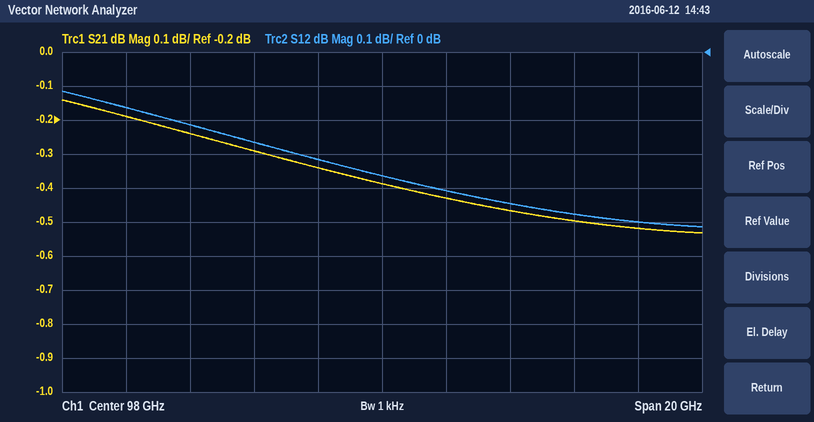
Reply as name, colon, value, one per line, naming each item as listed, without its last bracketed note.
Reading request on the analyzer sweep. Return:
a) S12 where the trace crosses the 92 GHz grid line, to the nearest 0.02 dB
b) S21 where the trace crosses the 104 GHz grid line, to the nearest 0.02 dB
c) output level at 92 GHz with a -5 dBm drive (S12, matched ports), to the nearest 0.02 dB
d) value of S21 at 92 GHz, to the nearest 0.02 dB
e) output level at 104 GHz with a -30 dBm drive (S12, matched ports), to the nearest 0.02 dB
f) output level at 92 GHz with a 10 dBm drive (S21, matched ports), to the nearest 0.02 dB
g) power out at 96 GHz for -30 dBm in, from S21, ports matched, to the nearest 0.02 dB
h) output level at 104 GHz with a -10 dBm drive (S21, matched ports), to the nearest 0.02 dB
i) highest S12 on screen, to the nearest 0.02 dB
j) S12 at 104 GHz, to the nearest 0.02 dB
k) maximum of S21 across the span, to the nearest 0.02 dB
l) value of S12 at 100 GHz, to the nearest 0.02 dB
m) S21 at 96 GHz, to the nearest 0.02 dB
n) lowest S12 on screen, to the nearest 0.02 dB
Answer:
S12 where the trace crosses the 92 GHz grid line, to the nearest 0.02 dB: -0.22 dB
S21 where the trace crosses the 104 GHz grid line, to the nearest 0.02 dB: -0.50 dB
output level at 92 GHz with a -5 dBm drive (S12, matched ports), to the nearest 0.02 dB: -5.22 dBm
value of S21 at 92 GHz, to the nearest 0.02 dB: -0.24 dB
output level at 104 GHz with a -30 dBm drive (S12, matched ports), to the nearest 0.02 dB: -30.48 dBm
output level at 92 GHz with a 10 dBm drive (S21, matched ports), to the nearest 0.02 dB: 9.76 dBm
power out at 96 GHz for -30 dBm in, from S21, ports matched, to the nearest 0.02 dB: -30.34 dBm
output level at 104 GHz with a -10 dBm drive (S21, matched ports), to the nearest 0.02 dB: -10.50 dBm
highest S12 on screen, to the nearest 0.02 dB: -0.12 dB
S12 at 104 GHz, to the nearest 0.02 dB: -0.48 dB
maximum of S21 across the span, to the nearest 0.02 dB: -0.14 dB
value of S12 at 100 GHz, to the nearest 0.02 dB: -0.40 dB
S21 at 96 GHz, to the nearest 0.02 dB: -0.34 dB
lowest S12 on screen, to the nearest 0.02 dB: -0.52 dB
